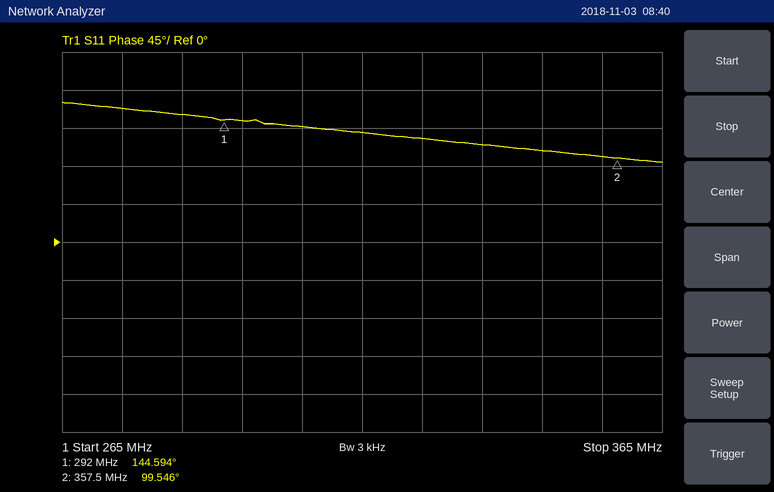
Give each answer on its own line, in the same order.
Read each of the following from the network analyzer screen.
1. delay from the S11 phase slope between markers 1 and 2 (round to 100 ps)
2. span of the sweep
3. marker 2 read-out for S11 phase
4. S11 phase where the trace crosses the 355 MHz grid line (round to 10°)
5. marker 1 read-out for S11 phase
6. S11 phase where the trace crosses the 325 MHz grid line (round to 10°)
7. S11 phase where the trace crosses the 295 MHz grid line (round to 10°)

1.9 ns
100 MHz
99.546°
100°
144.594°
120°
140°
